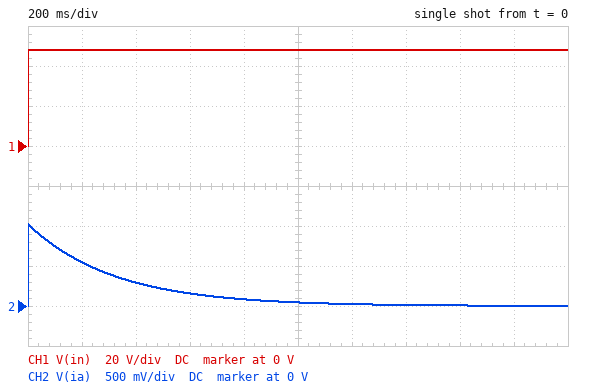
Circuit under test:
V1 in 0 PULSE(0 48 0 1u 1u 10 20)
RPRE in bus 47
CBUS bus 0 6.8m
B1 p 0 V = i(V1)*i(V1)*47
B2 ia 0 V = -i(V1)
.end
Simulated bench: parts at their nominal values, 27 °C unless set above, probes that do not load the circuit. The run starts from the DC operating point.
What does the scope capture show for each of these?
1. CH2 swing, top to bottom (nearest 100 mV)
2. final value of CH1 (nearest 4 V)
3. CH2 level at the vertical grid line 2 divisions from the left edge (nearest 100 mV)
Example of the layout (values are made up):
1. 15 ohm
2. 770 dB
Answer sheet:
1. 1.0 V
2. 48 V
3. 300 mV
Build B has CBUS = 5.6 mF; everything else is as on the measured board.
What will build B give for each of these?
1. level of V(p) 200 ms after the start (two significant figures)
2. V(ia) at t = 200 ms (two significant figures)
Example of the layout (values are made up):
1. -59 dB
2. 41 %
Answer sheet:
1. 11 V
2. 480 mV
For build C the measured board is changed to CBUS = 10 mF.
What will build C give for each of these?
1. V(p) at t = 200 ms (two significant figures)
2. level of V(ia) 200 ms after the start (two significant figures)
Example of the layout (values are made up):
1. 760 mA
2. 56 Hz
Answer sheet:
1. 21 V
2. 670 mV
